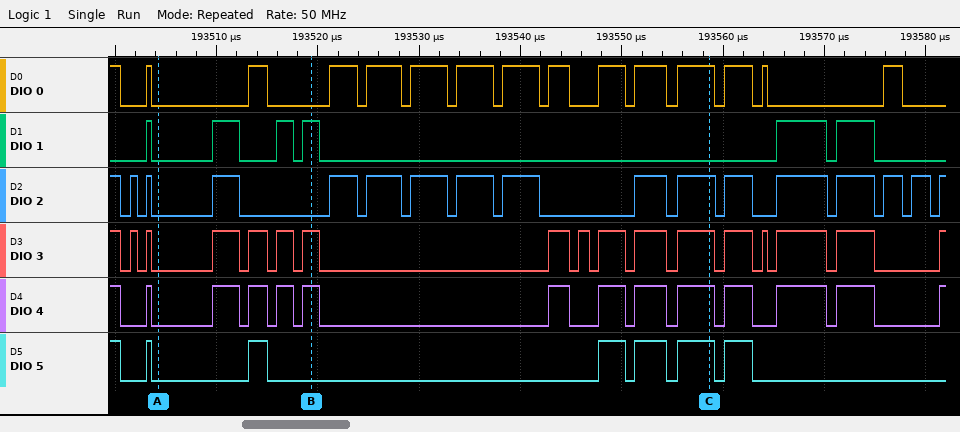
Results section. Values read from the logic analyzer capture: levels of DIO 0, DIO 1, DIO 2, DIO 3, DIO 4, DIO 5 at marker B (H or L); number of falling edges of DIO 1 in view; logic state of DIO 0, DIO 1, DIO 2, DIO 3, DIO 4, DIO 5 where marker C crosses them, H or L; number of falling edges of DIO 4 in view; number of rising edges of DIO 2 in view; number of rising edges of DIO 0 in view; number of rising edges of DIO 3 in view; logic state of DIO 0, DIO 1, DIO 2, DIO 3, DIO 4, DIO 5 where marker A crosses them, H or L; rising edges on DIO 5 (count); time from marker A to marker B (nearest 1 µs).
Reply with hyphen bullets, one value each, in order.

- DIO 0=L, DIO 1=H, DIO 2=L, DIO 3=H, DIO 4=H, DIO 5=L
- 6
- DIO 0=H, DIO 1=L, DIO 2=H, DIO 3=H, DIO 4=H, DIO 5=H
- 13
- 16
- 14
- 16
- DIO 0=L, DIO 1=L, DIO 2=L, DIO 3=L, DIO 4=L, DIO 5=L
- 6
- 15 µs
